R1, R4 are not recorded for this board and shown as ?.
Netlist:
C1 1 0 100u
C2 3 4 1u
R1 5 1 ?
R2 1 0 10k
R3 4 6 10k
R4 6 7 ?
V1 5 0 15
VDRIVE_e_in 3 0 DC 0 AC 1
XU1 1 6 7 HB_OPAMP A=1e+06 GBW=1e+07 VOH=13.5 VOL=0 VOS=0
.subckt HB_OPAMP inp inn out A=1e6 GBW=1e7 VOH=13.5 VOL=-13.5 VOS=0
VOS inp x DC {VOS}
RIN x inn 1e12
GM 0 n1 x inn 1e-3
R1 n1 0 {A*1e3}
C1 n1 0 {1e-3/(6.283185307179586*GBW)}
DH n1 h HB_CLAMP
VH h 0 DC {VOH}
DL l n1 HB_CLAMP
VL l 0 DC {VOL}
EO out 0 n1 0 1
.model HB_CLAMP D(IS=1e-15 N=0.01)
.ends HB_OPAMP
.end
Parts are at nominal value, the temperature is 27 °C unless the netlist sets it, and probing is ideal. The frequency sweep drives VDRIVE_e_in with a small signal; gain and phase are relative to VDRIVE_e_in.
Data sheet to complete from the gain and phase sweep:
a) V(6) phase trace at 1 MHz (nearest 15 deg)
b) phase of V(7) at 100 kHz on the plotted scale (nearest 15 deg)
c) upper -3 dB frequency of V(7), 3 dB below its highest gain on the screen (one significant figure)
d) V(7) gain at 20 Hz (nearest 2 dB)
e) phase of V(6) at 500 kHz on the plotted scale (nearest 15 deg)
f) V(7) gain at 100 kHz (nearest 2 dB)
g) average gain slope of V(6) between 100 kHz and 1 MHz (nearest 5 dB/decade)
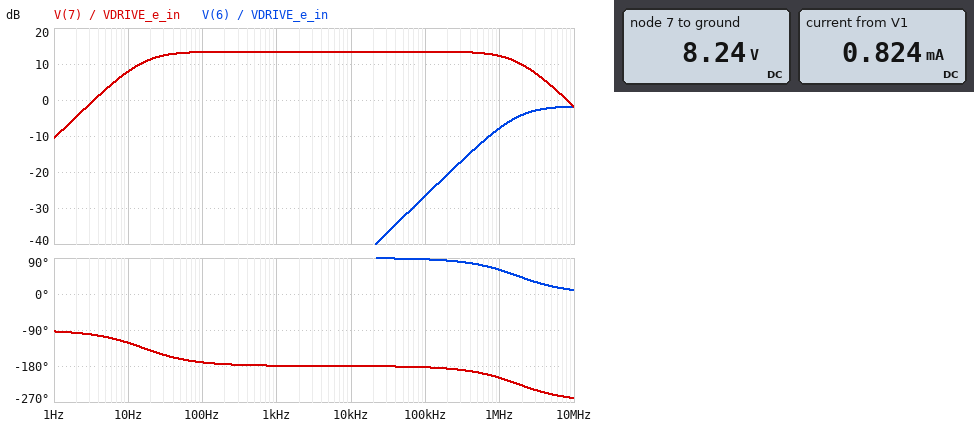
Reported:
60 deg
-180 deg
2 MHz
12 dB
75 deg
14 dB
20 dB/decade
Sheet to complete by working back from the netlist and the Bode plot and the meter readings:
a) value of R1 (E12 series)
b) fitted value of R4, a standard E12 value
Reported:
8.2 kΩ
47 kΩ
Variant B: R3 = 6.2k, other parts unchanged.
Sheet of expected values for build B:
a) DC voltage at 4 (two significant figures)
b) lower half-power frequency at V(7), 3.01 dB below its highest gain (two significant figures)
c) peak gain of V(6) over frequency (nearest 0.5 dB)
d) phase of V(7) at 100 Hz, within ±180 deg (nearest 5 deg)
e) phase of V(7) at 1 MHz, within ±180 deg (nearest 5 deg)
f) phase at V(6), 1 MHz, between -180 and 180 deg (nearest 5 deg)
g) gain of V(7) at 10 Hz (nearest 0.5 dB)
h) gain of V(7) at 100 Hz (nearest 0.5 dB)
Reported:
8.2 V
26 Hz
-1.0 dB
-165 deg
140 deg
50 deg
9.0 dB
17.5 dB
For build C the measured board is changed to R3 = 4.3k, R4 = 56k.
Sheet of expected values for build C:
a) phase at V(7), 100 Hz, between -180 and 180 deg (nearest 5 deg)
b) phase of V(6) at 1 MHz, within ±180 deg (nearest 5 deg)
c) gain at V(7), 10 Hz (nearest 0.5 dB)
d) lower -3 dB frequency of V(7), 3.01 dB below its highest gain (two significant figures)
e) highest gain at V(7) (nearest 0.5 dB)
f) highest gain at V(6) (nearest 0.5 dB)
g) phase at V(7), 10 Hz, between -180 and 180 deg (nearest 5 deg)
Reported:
-160 deg
35 deg
10.5 dB
37 Hz
22.5 dB
-0.5 dB
-105 deg
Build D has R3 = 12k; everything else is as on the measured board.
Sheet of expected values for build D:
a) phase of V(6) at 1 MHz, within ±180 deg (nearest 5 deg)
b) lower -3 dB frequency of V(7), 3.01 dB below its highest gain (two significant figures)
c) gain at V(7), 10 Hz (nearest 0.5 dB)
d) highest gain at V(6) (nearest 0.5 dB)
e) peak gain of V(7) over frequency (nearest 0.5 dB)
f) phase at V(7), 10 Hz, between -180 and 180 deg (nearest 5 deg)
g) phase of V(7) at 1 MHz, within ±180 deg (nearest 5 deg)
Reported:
65 deg
13 Hz
7.5 dB
-2.0 dB
12.0 dB
-125 deg
155 deg
